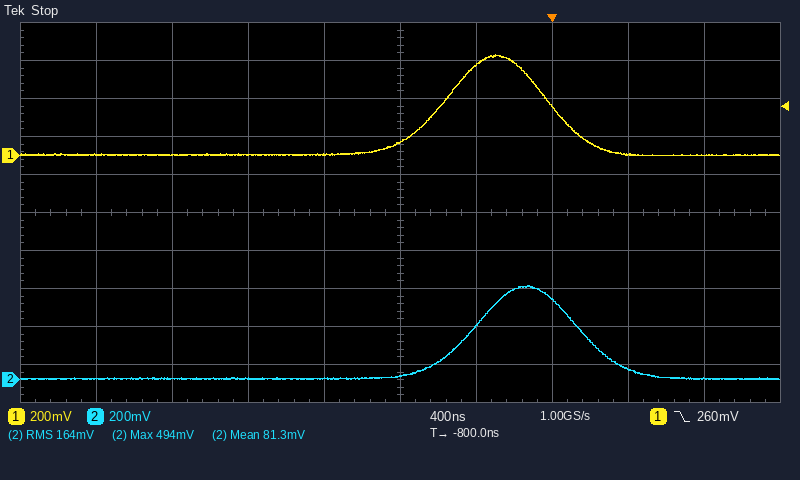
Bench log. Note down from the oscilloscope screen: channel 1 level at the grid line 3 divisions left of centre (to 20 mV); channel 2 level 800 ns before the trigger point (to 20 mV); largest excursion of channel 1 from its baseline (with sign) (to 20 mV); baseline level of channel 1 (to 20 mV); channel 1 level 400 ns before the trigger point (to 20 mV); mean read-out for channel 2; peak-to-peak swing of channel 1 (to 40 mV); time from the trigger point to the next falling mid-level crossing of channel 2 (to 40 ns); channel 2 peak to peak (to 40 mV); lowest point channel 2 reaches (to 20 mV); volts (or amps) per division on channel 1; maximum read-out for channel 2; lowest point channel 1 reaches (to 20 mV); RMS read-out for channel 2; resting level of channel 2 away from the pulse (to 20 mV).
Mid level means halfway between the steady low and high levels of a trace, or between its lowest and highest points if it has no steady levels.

0 mV
20 mV
+520 mV
0 mV
480 mV
81.3 mV
520 mV
160 ns
480 mV
0 mV
200 mV
494 mV
0 mV
164 mV
0 mV
